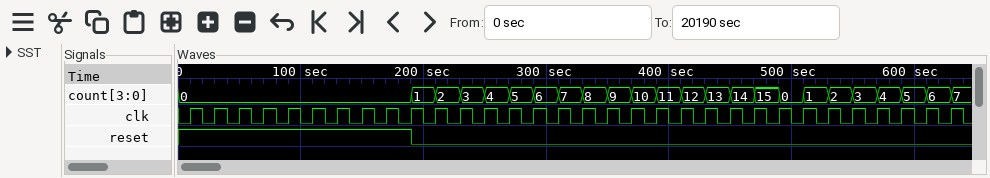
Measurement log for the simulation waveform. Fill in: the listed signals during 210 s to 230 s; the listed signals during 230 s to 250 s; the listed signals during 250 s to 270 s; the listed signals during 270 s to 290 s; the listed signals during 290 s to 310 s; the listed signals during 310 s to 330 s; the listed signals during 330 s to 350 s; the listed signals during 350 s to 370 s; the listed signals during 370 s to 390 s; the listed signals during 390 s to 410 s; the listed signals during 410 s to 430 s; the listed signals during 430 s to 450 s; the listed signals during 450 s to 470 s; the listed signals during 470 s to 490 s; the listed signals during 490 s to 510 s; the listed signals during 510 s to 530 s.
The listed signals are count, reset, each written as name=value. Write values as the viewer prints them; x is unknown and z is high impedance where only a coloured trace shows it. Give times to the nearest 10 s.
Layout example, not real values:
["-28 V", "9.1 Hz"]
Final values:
["count=2, reset=0", "count=3, reset=0", "count=4, reset=0", "count=5, reset=0", "count=6, reset=0", "count=7, reset=0", "count=8, reset=0", "count=9, reset=0", "count=10, reset=0", "count=11, reset=0", "count=12, reset=0", "count=13, reset=0", "count=14, reset=0", "count=15, reset=0", "count=0, reset=0", "count=1, reset=0"]
